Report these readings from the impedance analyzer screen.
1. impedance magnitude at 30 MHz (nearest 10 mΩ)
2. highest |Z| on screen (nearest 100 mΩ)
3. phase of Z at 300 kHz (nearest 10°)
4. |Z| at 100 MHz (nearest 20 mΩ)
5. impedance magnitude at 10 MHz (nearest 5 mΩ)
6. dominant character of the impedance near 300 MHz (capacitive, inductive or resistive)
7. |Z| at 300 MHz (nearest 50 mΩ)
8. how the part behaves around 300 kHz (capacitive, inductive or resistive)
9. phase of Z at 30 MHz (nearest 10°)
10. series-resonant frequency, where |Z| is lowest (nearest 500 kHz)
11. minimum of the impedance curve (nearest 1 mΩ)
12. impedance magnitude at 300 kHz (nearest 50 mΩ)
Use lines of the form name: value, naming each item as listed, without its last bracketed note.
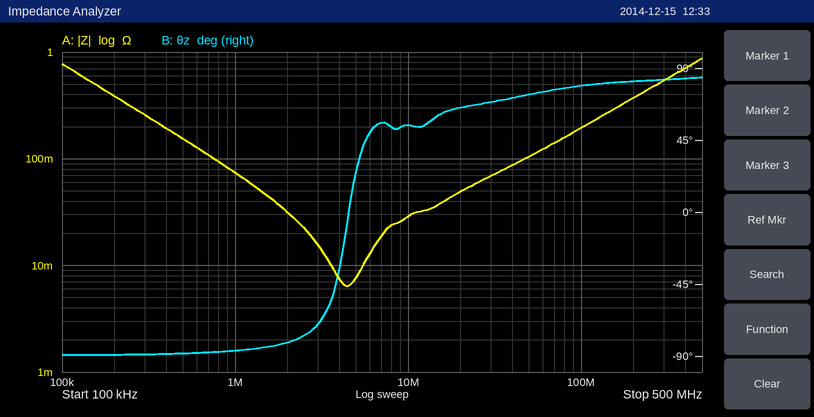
impedance magnitude at 30 MHz: 70 mΩ
highest |Z| on screen: 900 mΩ
phase of Z at 300 kHz: -90°
|Z| at 100 MHz: 200 mΩ
impedance magnitude at 10 MHz: 30 mΩ
dominant character of the impedance near 300 MHz: inductive
|Z| at 300 MHz: 550 mΩ
how the part behaves around 300 kHz: capacitive
phase of Z at 30 MHz: 70°
series-resonant frequency, where |Z| is lowest: 4.5 MHz
minimum of the impedance curve: 6 mΩ
impedance magnitude at 300 kHz: 250 mΩ
